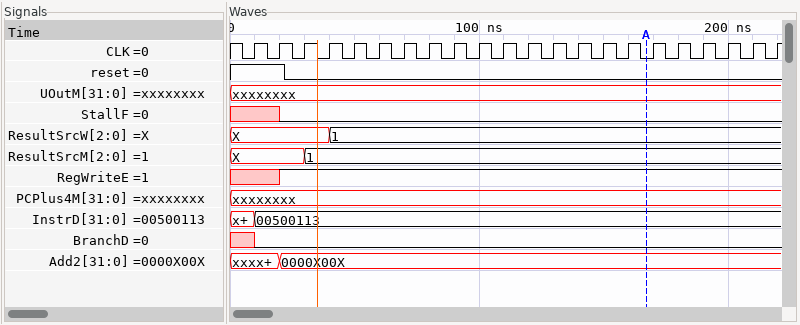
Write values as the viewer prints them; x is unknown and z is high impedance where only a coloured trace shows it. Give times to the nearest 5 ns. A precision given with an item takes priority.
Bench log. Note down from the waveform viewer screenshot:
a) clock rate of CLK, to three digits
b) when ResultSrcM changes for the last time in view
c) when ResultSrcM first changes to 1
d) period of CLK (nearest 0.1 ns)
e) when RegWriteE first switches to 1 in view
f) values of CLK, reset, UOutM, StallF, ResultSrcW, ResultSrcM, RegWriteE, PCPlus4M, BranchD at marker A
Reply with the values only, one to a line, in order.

100 MHz
30 ns
30 ns
10 ns
20 ns
CLK=0, reset=0, UOutM=xxxxxxxx, StallF=0, ResultSrcW=1, ResultSrcM=1, RegWriteE=1, PCPlus4M=xxxxxxxx, BranchD=0
